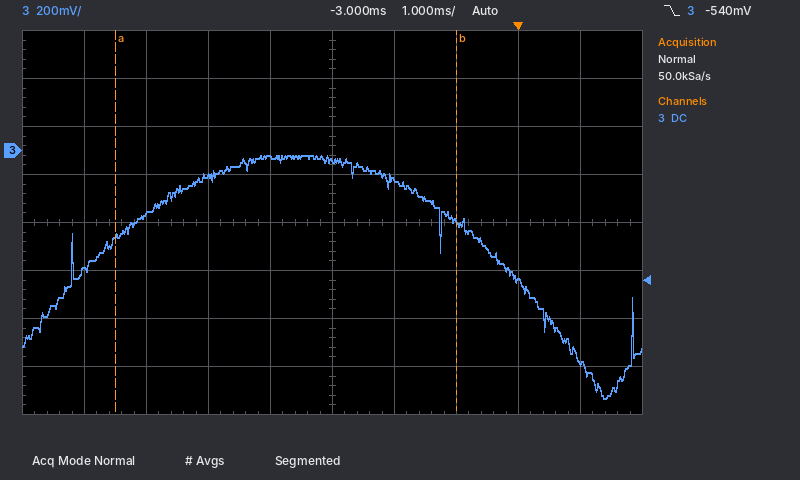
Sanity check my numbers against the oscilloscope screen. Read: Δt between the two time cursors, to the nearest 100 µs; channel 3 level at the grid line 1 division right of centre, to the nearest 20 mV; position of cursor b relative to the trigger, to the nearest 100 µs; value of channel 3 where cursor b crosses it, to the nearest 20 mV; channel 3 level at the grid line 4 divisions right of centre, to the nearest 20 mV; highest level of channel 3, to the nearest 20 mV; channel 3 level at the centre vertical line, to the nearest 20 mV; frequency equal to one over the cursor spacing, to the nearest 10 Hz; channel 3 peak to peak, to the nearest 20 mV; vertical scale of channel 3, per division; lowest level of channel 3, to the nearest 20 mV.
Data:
5.5 ms
-120 mV
-1.0 ms
-300 mV
-880 mV
-20 mV
-40 mV
180 Hz
1.02 V
200 mV
-1.04 V
